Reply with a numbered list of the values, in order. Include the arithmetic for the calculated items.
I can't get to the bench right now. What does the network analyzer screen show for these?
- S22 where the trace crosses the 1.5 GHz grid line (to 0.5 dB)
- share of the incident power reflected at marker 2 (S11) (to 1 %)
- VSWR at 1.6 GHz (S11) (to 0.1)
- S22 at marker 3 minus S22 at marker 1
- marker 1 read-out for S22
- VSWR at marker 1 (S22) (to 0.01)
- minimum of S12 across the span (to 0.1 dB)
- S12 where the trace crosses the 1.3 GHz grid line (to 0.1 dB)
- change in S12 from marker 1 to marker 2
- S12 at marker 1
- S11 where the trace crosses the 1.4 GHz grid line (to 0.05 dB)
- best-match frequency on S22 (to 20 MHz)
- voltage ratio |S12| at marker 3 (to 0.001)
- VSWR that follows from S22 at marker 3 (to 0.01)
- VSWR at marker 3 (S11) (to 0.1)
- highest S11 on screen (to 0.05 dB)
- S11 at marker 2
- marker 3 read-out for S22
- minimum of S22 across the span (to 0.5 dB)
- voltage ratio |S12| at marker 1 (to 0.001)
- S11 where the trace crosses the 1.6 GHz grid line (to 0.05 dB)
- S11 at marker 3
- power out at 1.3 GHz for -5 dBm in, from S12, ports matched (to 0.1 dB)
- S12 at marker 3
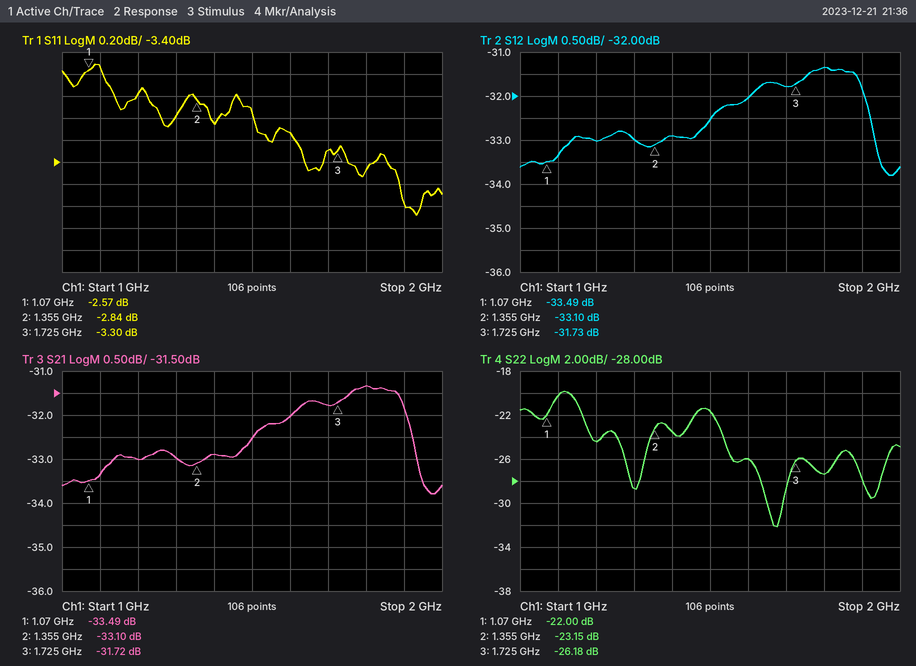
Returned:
1. -21.5 dB
2. 10^(-2.84/10) ≈ 52 %
3. |Γ| = 10^(-3.15/20) = 0.6958; VSWR = (1 + 0.6958)/(1 − 0.6958) ≈ 5.6
4. -26.18 − (-22) = -4.18 dB
5. -22.00 dB
6. (1 + 0.0794)/(1 − 0.0794) ≈ 1.17
7. -33.8 dB
8. -33.0 dB
9. -33.1 − (-33.49) = 0.39 dB
10. -33.49 dB
11. -3.05 dB
12. 1.68 GHz
13. 10^(-31.73/20) ≈ 0.026
14. (1 + 0.0491)/(1 − 0.0491) ≈ 1.10
15. (1 + 0.6839)/(1 − 0.6839) ≈ 5.3
16. -2.50 dB
17. -2.84 dB
18. -26.18 dB
19. -32.0 dB
20. 10^(-33.49/20) ≈ 0.021
21. -3.15 dB
22. -3.30 dB
23. -5 dBm + (-33.0 dB) = -38.0 dBm
24. -31.73 dB
